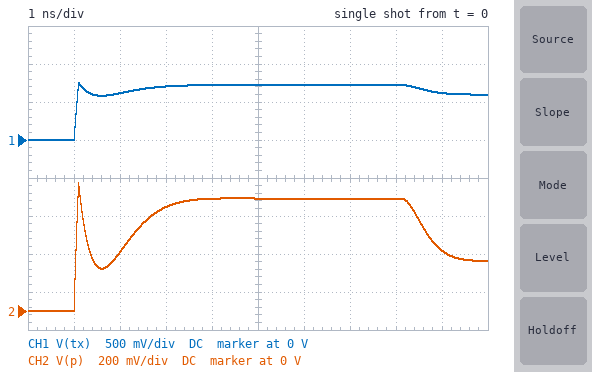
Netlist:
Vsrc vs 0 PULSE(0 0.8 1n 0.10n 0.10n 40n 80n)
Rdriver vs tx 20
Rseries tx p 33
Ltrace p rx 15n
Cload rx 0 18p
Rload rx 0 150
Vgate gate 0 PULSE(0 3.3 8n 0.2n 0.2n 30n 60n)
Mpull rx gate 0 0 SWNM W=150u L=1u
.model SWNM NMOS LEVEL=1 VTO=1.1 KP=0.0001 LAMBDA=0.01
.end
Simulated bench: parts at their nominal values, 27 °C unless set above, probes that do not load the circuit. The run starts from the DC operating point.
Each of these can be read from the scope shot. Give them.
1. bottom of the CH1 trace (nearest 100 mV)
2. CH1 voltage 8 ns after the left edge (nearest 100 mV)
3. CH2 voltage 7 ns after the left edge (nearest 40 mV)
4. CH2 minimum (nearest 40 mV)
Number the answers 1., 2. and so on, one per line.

1. 0 V
2. 700 mV
3. 600 mV
4. 0 V
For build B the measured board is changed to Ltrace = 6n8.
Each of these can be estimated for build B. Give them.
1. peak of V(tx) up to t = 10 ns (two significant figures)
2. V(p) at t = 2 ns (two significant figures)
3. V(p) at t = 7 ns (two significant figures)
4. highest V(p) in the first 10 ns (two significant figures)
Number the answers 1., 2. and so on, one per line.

1. 720 mV
2. 390 mV
3. 590 mV
4. 590 mV
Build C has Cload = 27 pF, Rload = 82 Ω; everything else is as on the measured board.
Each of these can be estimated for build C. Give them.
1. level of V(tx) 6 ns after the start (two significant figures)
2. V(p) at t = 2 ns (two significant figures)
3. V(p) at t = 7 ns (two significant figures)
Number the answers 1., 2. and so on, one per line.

1. 680 mV
2. 220 mV
3. 490 mV
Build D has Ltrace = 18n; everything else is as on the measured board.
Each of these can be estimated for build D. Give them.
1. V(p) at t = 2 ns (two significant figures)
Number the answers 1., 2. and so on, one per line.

1. 290 mV
